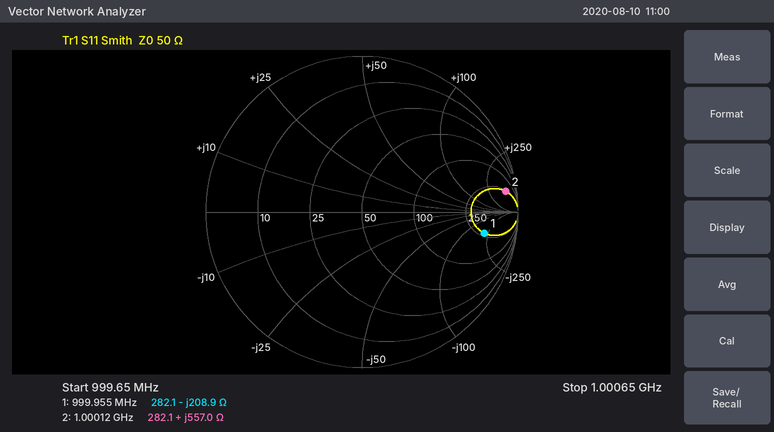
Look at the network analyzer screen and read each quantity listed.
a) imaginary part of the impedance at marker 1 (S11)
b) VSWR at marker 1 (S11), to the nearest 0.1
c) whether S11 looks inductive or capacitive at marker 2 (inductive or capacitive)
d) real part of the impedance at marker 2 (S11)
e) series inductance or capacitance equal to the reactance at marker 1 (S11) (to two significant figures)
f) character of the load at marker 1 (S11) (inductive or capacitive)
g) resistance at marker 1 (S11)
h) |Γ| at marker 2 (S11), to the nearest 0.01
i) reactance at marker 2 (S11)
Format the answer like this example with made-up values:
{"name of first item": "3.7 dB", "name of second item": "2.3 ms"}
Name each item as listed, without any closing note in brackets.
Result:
{"imaginary part of the impedance at marker 1": "-208.9 Ω", "VSWR at marker 1 (S11), to the nearest 0.1": "8.8", "whether S11 looks inductive or capacitive at marker 2": "inductive", "real part of the impedance at marker 2": "282.1 Ω", "series inductance or capacitance equal to the reactance at marker 1 (S11)": "760 fF", "character of the load at marker 1 (S11)": "capacitive", "resistance at marker 1": "282.1 Ω", "|Γ| at marker 2 (S11), to the nearest 0.01": "0.93", "reactance at marker 2": "+557.0 Ω"}
